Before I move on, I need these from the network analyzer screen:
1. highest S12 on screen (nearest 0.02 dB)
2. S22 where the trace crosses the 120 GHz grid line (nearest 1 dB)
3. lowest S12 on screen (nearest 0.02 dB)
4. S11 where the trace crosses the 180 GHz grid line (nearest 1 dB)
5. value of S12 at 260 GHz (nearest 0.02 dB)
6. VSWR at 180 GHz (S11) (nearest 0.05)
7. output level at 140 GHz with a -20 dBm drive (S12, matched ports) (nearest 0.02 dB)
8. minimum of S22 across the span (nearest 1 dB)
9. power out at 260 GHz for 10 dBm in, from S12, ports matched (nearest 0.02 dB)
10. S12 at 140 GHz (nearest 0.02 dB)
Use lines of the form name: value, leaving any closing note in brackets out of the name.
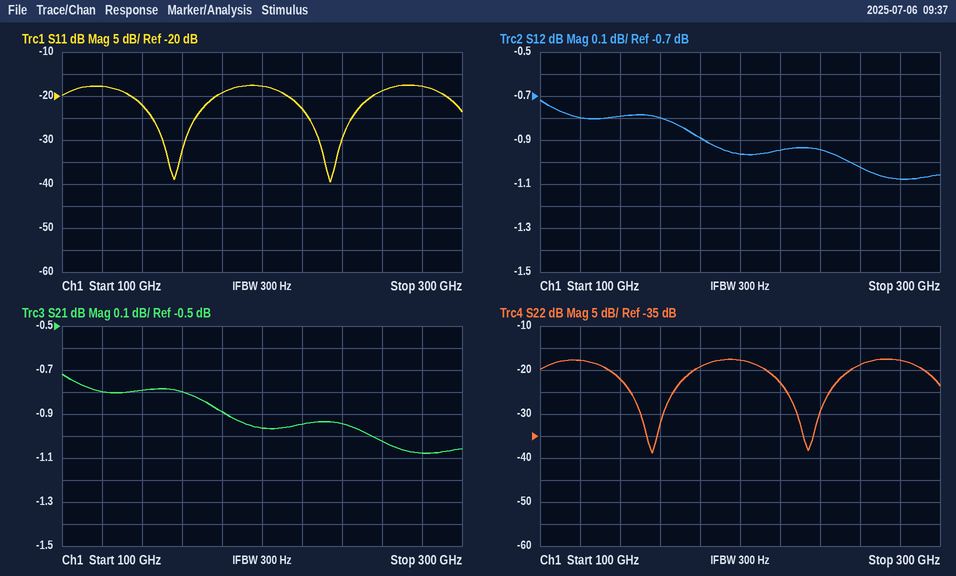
highest S12 on screen: -0.72 dB
S22 where the trace crosses the 120 GHz grid line: -18 dB
lowest S12 on screen: -1.08 dB
S11 where the trace crosses the 180 GHz grid line: -19 dB
value of S12 at 260 GHz: -1.02 dB
VSWR at 180 GHz (S11): 1.25
output level at 140 GHz with a -20 dBm drive (S12, matched ports): -20.80 dBm
minimum of S22 across the span: -39 dB
power out at 260 GHz for 10 dBm in, from S12, ports matched: 8.98 dBm
S12 at 140 GHz: -0.80 dB
